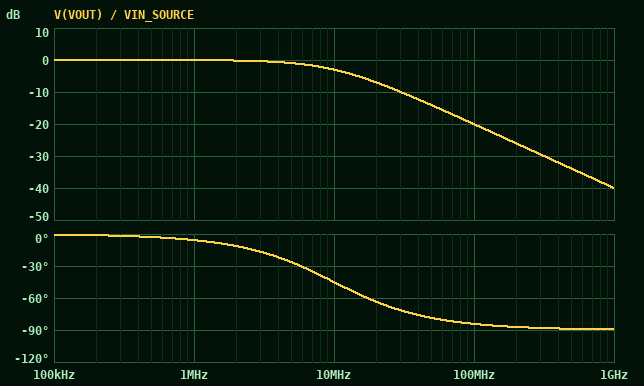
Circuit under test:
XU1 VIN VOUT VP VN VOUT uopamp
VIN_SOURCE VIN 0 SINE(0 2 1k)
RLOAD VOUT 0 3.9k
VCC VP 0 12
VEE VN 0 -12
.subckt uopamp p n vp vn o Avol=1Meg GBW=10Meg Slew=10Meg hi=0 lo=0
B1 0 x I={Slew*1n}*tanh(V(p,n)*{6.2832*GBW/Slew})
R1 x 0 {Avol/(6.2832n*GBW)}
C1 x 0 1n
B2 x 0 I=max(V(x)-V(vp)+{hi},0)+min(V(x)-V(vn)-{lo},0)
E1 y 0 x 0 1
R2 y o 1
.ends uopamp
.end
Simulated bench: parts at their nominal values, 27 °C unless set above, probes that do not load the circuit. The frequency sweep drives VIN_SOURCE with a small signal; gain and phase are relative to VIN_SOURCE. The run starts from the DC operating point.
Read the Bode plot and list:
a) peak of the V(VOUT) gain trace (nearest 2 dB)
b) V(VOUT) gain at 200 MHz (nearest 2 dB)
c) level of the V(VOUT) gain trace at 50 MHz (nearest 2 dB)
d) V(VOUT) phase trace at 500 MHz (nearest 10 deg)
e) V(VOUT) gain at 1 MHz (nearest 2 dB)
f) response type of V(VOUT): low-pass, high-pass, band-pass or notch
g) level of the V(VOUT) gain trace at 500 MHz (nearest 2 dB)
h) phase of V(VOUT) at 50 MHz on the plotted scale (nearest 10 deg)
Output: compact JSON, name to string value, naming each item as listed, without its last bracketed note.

{"peak of the V(VOUT) gain trace": "0 dB", "V(VOUT) gain at 200 MHz": "-26 dB", "level of the V(VOUT) gain trace at 50 MHz": "-14 dB", "V(VOUT) phase trace at 500 MHz": "-90 deg", "V(VOUT) gain at 1 MHz": "0 dB", "response type of V(VOUT): low-pass, high-pass, band-pass or notch": "low-pass", "level of the V(VOUT) gain trace at 500 MHz": "-34 dB", "phase of V(VOUT) at 50 MHz on the plotted scale": "-80 deg"}
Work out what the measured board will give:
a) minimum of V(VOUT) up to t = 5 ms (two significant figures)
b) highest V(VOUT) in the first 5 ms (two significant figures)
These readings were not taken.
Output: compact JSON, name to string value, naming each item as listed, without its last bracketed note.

{"minimum of V(VOUT) up to t = 5 ms": "-2.0 V", "highest V(VOUT) in the first 5 ms": "2.0 V"}
